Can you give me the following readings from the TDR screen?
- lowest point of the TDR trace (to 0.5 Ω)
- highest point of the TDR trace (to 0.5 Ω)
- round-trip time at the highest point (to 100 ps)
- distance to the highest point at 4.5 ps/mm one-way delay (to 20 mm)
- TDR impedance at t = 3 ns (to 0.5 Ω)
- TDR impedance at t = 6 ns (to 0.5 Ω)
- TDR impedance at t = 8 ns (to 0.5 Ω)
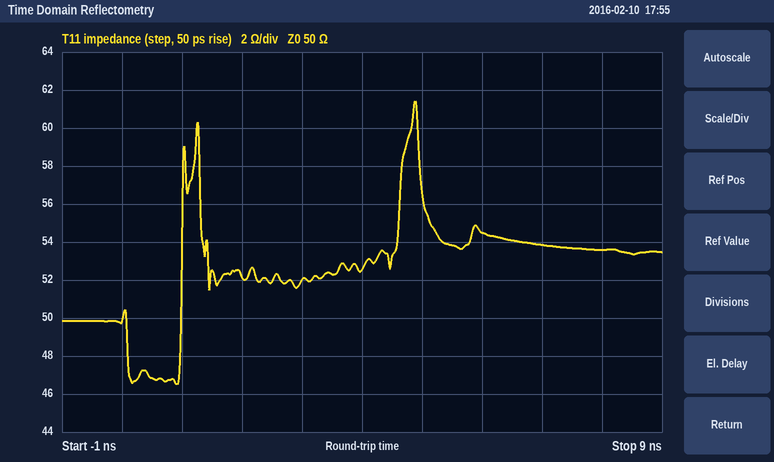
46.5 Ω
61.5 Ω
4.9 ns
540 mm
52.0 Ω
54.5 Ω
53.5 Ω
